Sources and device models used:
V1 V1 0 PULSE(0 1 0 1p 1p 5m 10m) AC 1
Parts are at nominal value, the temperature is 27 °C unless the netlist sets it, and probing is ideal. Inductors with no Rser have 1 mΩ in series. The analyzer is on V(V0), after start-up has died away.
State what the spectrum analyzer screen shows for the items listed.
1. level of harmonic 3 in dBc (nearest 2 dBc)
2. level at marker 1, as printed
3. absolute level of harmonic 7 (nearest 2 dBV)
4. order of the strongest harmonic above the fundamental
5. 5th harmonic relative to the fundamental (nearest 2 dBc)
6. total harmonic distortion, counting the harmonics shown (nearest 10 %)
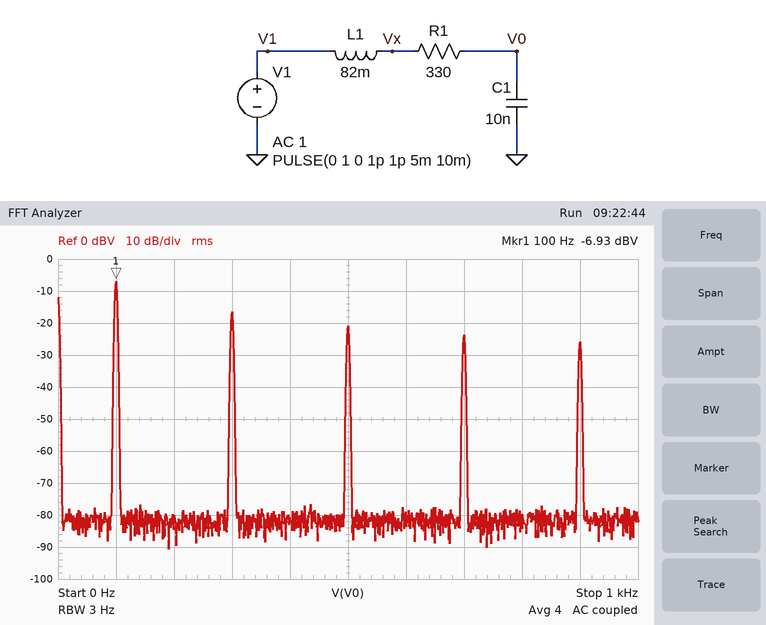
-10 dBc
-6.93 dBV
-24 dBV
3
-14 dBc
40 %
